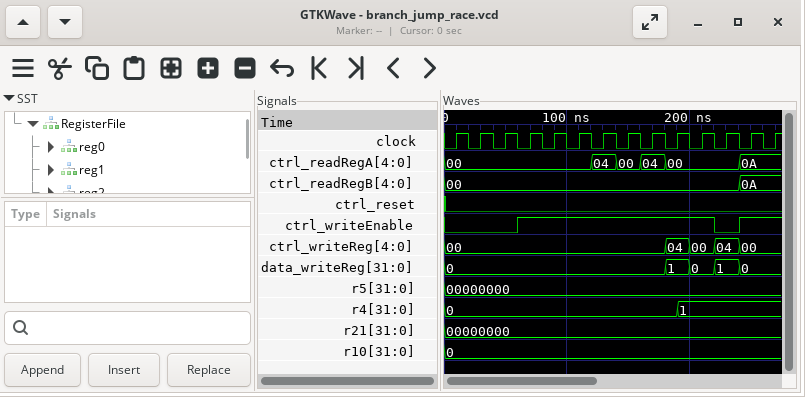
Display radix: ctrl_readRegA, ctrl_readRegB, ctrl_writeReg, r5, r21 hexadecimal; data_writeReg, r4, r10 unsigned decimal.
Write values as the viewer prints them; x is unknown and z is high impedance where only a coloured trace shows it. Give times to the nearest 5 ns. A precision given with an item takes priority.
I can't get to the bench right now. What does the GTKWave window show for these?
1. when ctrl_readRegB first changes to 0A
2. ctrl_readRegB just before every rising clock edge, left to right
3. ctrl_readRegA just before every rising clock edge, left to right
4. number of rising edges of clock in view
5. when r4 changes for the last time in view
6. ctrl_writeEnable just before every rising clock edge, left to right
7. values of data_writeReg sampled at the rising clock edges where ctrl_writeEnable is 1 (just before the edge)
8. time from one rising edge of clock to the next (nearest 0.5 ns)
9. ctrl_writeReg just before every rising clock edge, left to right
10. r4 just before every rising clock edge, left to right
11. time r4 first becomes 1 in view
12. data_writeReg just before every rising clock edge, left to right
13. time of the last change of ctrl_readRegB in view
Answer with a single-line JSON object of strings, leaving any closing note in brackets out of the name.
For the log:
{"when ctrl_readRegB first changes to 0A": "240 ns", "ctrl_readRegB just before every rising clock edge, left to right": "00, 00, 00, 00, 00, 00, 00, 00, 00, 00, 00, 00, 0A, 0A", "ctrl_readRegA just before every rising clock edge, left to right": "00, 00, 00, 00, 00, 00, 04, 00, 04, 00, 00, 00, 0A, 0A", "number of rising edges of clock in view": "14", "when r4 changes for the last time in view": "190 ns", "ctrl_writeEnable just before every rising clock edge, left to right": "0 0 0 1 1 1 1 1 1 1 1 0 1 1", "values of data_writeReg sampled at the rising clock edges where ctrl_writeEnable is 1": "0, 0, 0, 0, 0, 0, 1, 0, 0, 0", "time from one rising edge of clock to the next": "20 ns", "ctrl_writeReg just before every rising clock edge, left to right": "00, 00, 00, 00, 00, 00, 00, 00, 00, 04, 00, 04, 00, 00", "r4 just before every rising clock edge, left to right": "0, 0, 0, 0, 0, 0, 0, 0, 0, 0, 1, 1, 1, 1", "time r4 first becomes 1 in view": "190 ns", "data_writeReg just before every rising clock edge, left to right": "0, 0, 0, 0, 0, 0, 0, 0, 0, 1, 0, 1, 0, 0", "time of the last change of ctrl_readRegB in view": "240 ns"}
